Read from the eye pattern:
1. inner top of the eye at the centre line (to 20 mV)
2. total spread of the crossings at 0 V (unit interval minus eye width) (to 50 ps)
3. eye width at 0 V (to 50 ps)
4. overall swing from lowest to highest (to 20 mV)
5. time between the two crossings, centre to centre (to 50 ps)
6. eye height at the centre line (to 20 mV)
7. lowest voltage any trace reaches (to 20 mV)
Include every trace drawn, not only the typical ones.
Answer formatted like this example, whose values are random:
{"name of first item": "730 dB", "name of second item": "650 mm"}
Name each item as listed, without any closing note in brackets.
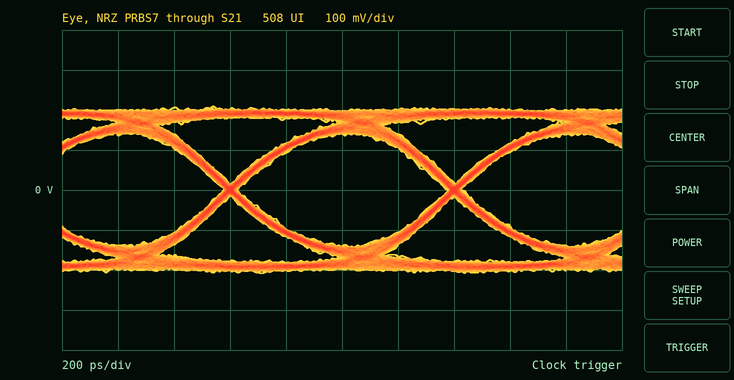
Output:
{"inner top of the eye at the centre line": "140 mV", "total spread of the crossings at 0 V (unit interval minus eye width)": "50 ps", "eye width at 0 V": "750 ps", "overall swing from lowest to highest": "420 mV", "time between the two crossings, centre to centre": "800 ps", "eye height at the centre line": "280 mV", "lowest voltage any trace reaches": "-200 mV"}
